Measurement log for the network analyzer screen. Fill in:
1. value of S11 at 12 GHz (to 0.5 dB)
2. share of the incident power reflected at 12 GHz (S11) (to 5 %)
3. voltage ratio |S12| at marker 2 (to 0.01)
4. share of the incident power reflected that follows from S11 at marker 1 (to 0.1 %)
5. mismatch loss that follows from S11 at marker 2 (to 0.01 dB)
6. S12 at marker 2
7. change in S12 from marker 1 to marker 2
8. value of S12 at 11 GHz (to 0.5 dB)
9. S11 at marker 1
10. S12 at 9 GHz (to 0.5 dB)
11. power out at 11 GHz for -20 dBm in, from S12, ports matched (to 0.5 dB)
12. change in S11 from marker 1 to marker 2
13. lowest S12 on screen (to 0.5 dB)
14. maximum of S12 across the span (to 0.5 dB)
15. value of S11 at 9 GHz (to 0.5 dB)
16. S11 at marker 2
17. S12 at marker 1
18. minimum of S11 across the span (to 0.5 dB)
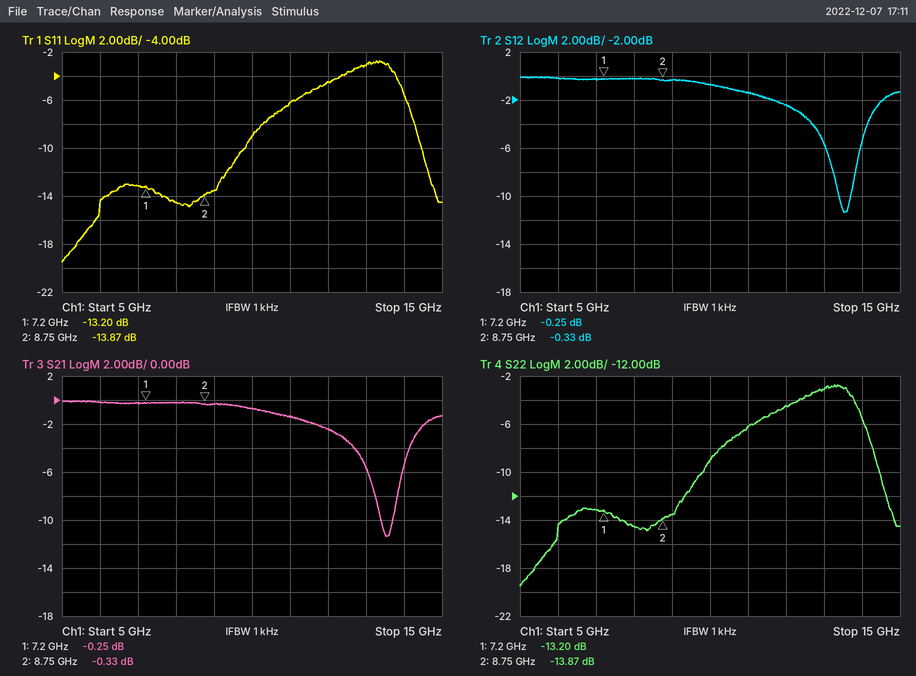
-4.5 dB
35 %
0.96
4.8 %
0.18 dB
-0.33 dB
-0.08 dB
-1.5 dB
-13.20 dB
-0.5 dB
-21.5 dBm
-0.67 dB
-11.5 dB
0.0 dB
-13.5 dB
-13.87 dB
-0.25 dB
-19.5 dB
